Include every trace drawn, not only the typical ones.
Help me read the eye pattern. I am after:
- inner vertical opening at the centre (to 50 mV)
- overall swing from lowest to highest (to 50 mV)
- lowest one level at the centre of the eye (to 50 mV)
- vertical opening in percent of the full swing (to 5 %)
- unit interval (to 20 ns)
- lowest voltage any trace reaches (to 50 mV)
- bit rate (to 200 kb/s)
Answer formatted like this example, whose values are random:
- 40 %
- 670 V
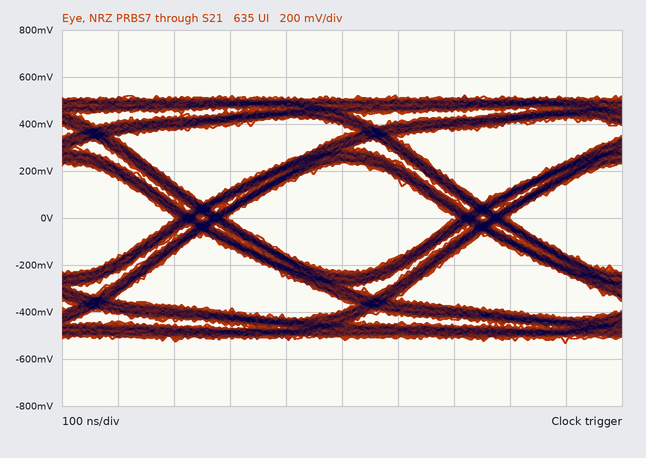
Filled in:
- 450 mV
- 1.05 V
- 250 mV
- 45 %
- 500 ns
- -550 mV
- 2.0 Mb/s
